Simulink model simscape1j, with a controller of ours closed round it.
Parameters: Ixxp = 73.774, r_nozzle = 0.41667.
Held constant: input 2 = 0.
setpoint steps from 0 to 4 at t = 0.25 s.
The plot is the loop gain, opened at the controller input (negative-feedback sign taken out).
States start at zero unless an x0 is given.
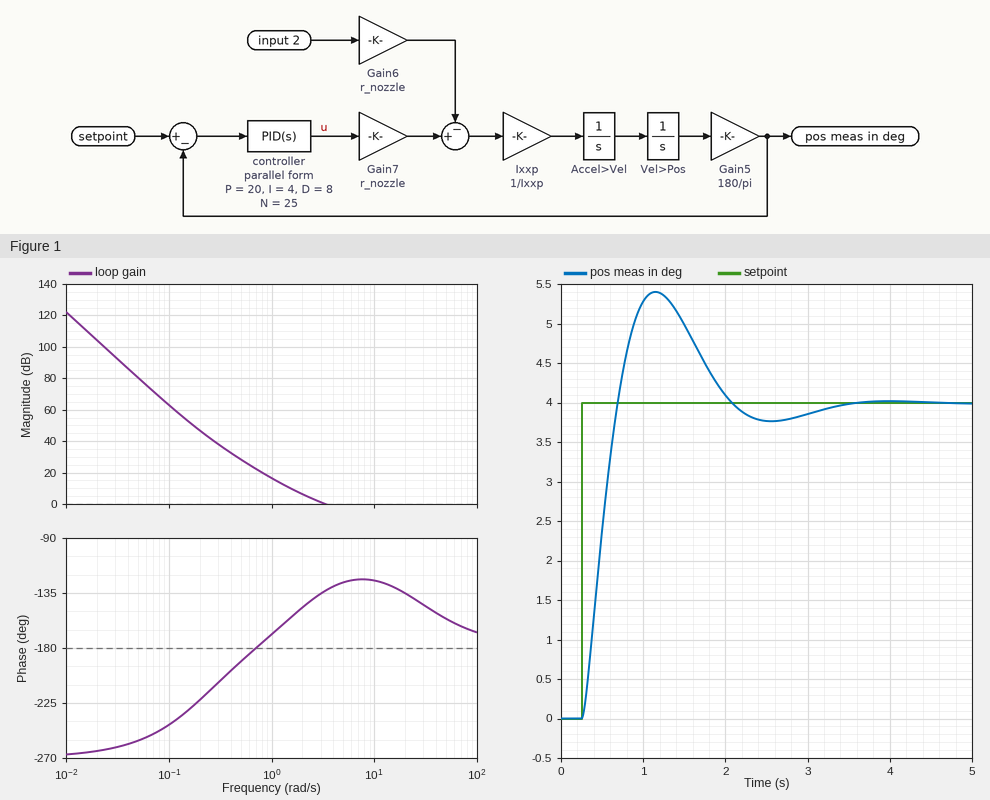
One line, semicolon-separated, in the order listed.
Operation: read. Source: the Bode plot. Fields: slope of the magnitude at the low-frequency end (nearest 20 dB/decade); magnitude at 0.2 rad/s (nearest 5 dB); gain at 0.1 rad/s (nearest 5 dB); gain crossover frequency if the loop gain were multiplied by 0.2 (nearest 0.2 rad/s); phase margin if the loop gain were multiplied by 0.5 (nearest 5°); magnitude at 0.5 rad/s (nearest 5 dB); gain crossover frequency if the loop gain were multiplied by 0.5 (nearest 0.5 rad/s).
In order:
-60 dB/decade; 45 dB; 65 dB; 1.2 rad/s; 35°; 30 dB; 2.0 rad/s
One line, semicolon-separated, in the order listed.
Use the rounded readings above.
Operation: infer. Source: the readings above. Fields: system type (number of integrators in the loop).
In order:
3
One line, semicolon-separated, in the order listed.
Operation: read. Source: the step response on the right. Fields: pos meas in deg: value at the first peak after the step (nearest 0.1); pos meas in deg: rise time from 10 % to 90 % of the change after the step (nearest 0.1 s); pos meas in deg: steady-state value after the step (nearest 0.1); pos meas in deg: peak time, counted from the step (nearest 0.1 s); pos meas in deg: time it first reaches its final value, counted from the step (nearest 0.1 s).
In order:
5.4; 0.3 s; 4.0; 0.9 s; 0.4 s
